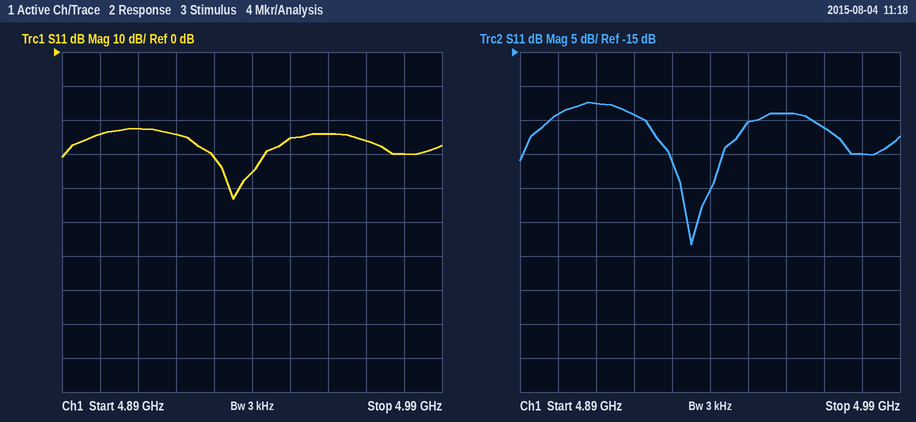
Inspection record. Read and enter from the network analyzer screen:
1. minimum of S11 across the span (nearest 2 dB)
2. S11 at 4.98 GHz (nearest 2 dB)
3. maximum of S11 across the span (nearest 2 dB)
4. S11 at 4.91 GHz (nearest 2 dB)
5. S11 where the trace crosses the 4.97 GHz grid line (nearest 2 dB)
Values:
-44 dB
-30 dB
-22 dB
-22 dB
-26 dB
